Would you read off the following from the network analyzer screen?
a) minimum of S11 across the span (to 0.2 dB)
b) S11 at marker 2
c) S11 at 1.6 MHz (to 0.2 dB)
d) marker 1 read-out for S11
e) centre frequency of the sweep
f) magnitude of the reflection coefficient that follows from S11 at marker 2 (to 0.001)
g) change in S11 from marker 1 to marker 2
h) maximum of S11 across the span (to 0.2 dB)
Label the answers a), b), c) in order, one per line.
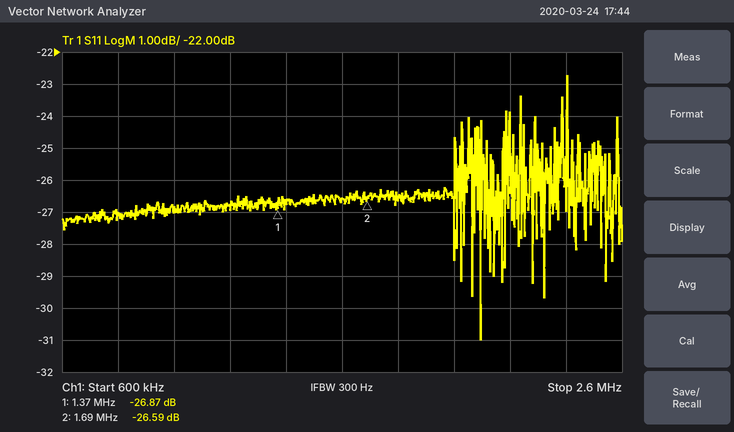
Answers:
a) -31.0 dB
b) -26.59 dB
c) -26.6 dB
d) -26.87 dB
e) 1.6 MHz
f) 0.047
g) 0.28 dB
h) -22.8 dB
